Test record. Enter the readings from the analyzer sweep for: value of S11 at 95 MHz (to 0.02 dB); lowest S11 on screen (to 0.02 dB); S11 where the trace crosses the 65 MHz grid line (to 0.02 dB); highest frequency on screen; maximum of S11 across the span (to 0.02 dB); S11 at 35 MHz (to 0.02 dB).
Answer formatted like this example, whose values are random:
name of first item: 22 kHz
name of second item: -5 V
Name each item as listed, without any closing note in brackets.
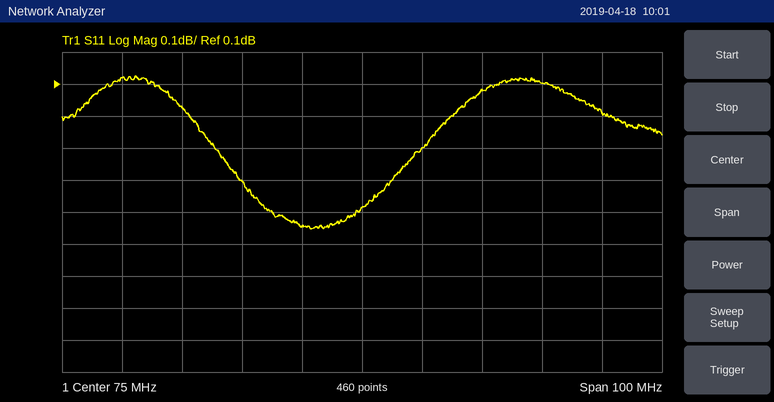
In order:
value of S11 at 95 MHz: 0.08 dB
lowest S11 on screen: -0.36 dB
S11 where the trace crosses the 65 MHz grid line: -0.34 dB
highest frequency on screen: 125 MHz
maximum of S11 across the span: 0.12 dB
S11 at 35 MHz: 0.12 dB
